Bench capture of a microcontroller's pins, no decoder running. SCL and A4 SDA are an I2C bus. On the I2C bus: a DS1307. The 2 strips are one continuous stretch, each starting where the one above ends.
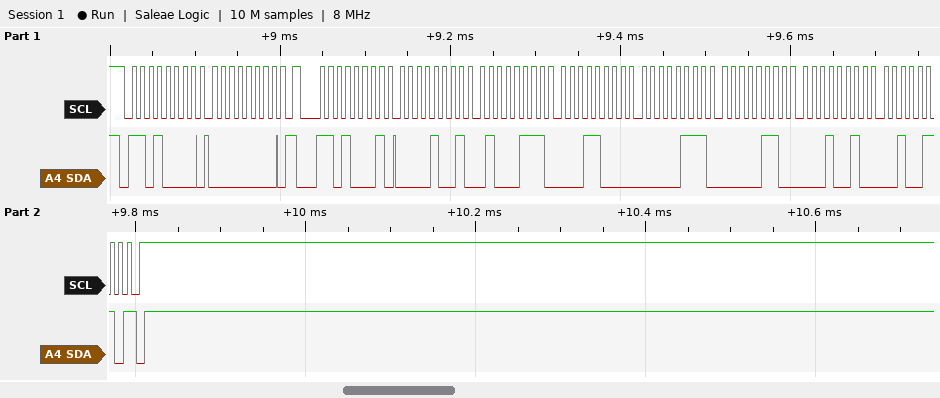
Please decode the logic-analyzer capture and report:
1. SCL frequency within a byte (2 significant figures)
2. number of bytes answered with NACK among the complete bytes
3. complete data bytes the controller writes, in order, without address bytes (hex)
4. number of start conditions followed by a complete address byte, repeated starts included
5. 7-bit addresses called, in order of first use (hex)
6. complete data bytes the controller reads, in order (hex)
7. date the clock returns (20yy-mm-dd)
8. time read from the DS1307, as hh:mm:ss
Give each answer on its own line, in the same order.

100 kHz
1
00
2
0x68
09 47 18 07 06 12 26
2026-12-06
18:47:09
